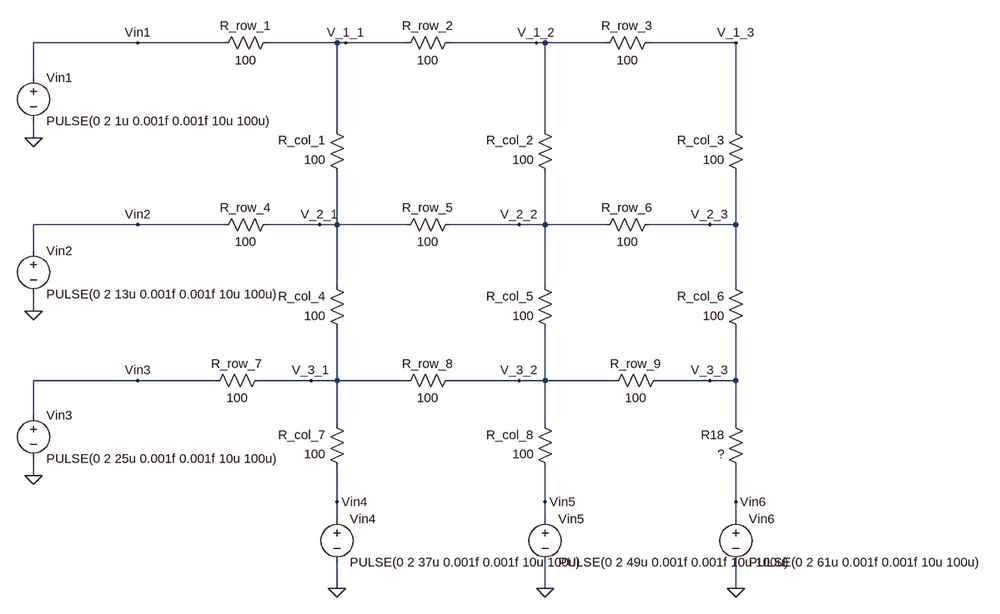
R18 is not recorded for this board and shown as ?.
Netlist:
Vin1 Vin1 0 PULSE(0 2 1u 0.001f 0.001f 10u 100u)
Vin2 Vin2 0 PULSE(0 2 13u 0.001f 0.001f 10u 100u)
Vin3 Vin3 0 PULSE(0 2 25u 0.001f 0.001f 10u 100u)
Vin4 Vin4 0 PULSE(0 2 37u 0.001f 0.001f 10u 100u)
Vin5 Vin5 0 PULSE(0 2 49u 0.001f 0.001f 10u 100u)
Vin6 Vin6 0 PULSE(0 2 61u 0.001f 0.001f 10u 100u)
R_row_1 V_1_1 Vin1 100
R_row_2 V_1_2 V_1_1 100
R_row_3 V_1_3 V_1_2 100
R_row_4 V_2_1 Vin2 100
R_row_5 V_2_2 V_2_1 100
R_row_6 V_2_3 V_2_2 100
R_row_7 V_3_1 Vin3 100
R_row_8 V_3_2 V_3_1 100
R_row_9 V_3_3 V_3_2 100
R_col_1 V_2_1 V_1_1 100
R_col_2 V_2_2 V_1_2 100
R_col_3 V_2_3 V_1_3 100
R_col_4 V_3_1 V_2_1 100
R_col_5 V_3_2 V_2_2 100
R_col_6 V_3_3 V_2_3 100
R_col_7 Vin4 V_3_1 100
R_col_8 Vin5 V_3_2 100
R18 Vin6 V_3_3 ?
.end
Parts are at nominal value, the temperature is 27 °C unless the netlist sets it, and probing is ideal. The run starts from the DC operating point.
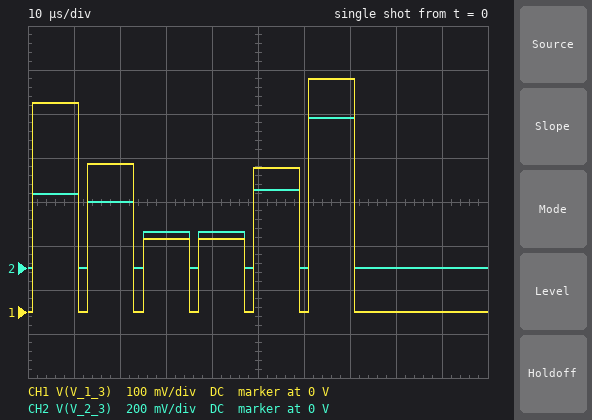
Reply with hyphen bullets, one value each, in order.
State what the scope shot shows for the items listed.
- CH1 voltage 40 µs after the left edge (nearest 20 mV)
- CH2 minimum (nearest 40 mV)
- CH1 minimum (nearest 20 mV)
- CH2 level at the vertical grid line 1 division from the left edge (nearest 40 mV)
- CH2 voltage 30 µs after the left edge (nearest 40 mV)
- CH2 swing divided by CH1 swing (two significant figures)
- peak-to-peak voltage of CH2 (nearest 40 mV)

- 160 mV
- 0 V
- 0 V
- 320 mV
- 160 mV
- 1.3
- 680 mV
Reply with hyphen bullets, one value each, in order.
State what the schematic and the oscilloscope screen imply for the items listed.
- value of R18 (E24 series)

- 82 Ω
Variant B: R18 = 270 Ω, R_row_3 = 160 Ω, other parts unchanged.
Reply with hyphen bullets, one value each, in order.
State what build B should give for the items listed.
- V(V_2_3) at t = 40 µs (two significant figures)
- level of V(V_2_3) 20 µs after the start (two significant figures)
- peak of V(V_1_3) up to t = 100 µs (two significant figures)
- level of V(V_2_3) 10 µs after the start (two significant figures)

- 210 mV
- 360 mV
- 490 mV
- 380 mV
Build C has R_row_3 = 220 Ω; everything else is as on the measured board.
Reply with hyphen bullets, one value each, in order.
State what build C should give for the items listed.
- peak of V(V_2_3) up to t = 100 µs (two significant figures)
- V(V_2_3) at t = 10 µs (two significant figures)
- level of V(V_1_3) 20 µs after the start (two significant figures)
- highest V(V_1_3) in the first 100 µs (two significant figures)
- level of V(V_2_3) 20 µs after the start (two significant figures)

- 710 mV
- 310 mV
- 320 mV
- 600 mV
- 290 mV
